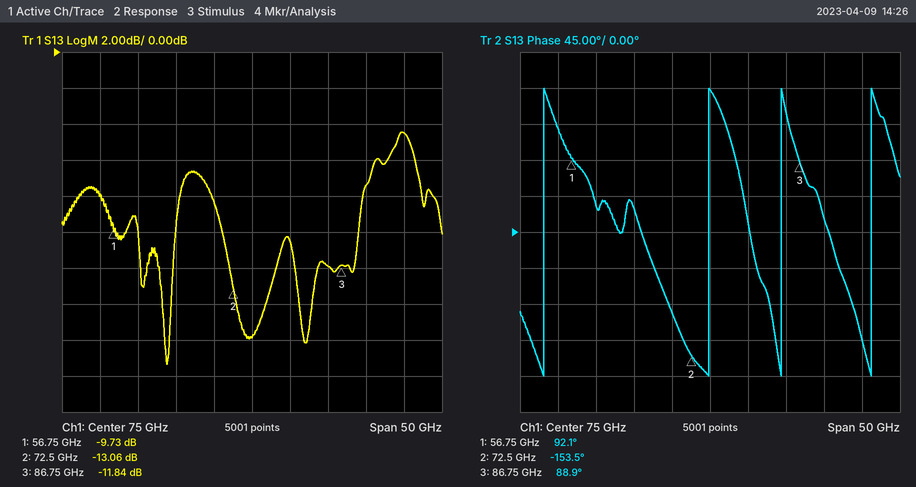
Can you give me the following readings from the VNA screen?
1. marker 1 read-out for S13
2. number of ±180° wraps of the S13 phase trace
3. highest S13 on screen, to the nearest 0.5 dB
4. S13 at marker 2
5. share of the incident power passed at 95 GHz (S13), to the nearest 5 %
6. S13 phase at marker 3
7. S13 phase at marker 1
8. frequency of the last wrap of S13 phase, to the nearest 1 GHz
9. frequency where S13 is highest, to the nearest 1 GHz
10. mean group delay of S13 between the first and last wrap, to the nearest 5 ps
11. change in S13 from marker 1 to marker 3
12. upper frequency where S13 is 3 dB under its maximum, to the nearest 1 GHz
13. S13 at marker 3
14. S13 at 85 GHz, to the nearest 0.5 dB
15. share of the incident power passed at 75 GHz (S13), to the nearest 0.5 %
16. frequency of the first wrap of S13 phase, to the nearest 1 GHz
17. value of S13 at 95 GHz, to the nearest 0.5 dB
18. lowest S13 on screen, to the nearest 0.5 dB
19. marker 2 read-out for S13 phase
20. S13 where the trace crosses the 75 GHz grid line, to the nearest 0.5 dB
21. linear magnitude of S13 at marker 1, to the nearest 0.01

-9.73 dB
4
-4.5 dB
-13.06 dB
35 %
88.9°
92.1°
96 GHz
95 GHz
70 ps
-2.11 dB
97 GHz
-11.84 dB
-12.0 dB
2.5 %
53 GHz
-4.5 dB
-17.5 dB
-153.5°
-16.0 dB
0.33
